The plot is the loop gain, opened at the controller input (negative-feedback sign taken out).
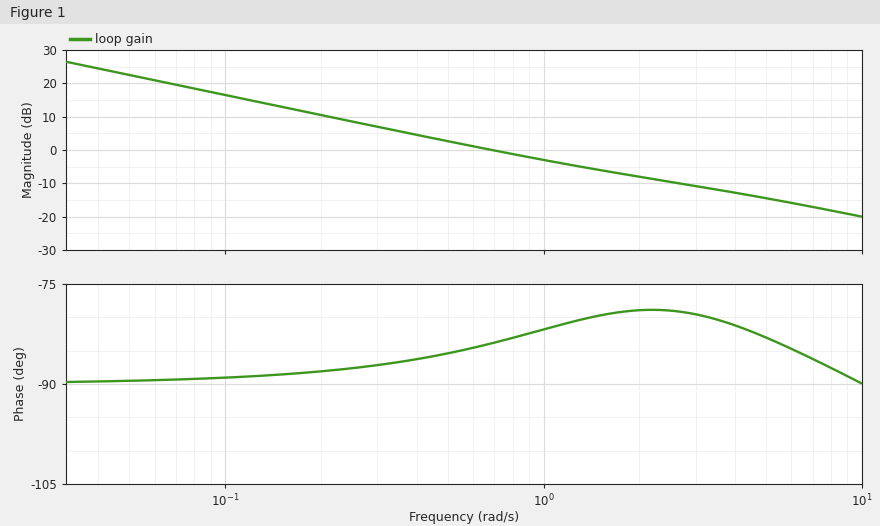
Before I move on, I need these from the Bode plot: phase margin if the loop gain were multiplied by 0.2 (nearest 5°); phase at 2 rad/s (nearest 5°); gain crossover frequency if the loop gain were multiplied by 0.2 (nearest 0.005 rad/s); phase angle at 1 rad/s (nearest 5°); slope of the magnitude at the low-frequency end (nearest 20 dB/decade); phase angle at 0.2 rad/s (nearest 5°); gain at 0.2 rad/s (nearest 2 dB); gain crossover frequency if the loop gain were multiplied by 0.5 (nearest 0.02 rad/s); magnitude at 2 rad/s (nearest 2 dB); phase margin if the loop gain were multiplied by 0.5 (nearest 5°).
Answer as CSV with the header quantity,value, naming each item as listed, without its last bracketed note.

quantity,value
phase margin if the loop gain were multiplied by 0.2,90°
phase at 2 rad/s,-80°
gain crossover frequency if the loop gain were multiplied by 0.2,0.135 rad/s
phase angle at 1 rad/s,-80°
slope of the magnitude at the low-frequency end,-20 dB/decade
phase angle at 0.2 rad/s,-90°
gain at 0.2 rad/s,10 dB
gain crossover frequency if the loop gain were multiplied by 0.5,0.34 rad/s
magnitude at 2 rad/s,-8 dB
phase margin if the loop gain were multiplied by 0.5,95°
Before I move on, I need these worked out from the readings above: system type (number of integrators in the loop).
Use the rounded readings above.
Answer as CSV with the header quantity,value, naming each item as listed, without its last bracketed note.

quantity,value
system type,1
